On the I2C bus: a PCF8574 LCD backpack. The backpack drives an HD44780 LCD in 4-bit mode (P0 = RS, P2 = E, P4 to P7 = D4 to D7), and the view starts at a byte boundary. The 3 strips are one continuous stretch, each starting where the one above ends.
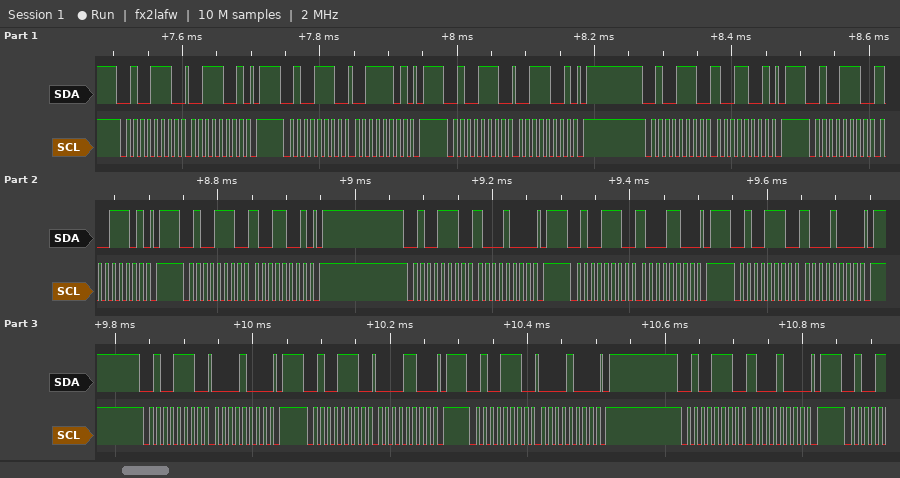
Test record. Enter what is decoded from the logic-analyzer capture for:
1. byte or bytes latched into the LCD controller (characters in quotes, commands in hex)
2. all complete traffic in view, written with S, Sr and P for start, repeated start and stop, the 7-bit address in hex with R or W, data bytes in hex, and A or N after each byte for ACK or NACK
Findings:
'9' 0x80
S 27W A 39 A P S 27W A 3D A P S 27W A 39 A P S 27W A 99 A P S 27W A 9D A P S 27W A 99 A P S 27W A 88 A P S 27W A 8C A P S 27W A 88 A P S 27W A 08 A P S 27W A 0C A P S 27W A 08 A P S 27W A 88 A P
